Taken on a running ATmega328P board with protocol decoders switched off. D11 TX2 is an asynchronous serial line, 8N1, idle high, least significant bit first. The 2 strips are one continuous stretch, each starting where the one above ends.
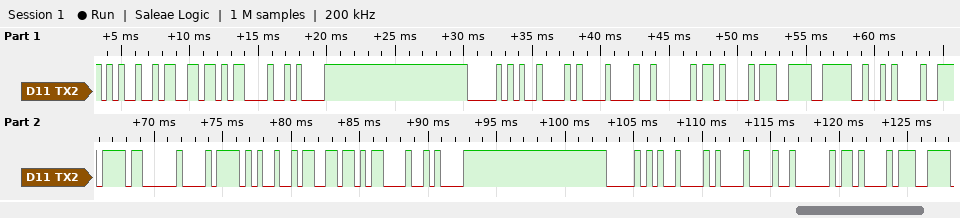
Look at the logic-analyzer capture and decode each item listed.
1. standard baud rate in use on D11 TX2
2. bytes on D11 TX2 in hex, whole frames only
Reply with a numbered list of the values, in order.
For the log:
1. 2400 baud
2. 0x25 0xB3 0x0D 0x0A 0x50 0x42 0x08 0x02 0x0B 0xE7 0x3E 0x0A 0xEE 0x03 0xE8 0x25 0xB3 0x0D 0x0A 0x50 0x42 0x08 0x02 0x0B 0xE7
